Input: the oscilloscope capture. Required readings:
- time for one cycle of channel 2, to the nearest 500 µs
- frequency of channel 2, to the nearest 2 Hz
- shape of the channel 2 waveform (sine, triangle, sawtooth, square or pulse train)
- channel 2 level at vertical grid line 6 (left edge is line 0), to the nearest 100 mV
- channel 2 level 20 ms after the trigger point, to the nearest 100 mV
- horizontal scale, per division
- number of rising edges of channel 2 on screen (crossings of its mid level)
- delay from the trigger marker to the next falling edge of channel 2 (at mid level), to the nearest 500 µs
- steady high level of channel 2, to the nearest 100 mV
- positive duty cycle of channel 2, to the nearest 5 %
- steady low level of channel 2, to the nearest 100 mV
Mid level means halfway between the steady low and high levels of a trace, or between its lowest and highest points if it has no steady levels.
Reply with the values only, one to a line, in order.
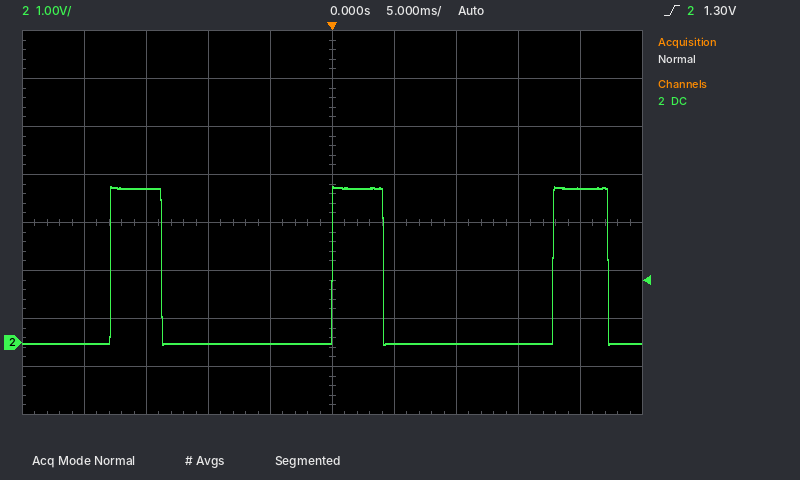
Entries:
18.0 ms
56 Hz
pulse train
0.0 V
3.2 V
5 ms
3
4.0 ms
3.2 V
25 %
0.0 V
